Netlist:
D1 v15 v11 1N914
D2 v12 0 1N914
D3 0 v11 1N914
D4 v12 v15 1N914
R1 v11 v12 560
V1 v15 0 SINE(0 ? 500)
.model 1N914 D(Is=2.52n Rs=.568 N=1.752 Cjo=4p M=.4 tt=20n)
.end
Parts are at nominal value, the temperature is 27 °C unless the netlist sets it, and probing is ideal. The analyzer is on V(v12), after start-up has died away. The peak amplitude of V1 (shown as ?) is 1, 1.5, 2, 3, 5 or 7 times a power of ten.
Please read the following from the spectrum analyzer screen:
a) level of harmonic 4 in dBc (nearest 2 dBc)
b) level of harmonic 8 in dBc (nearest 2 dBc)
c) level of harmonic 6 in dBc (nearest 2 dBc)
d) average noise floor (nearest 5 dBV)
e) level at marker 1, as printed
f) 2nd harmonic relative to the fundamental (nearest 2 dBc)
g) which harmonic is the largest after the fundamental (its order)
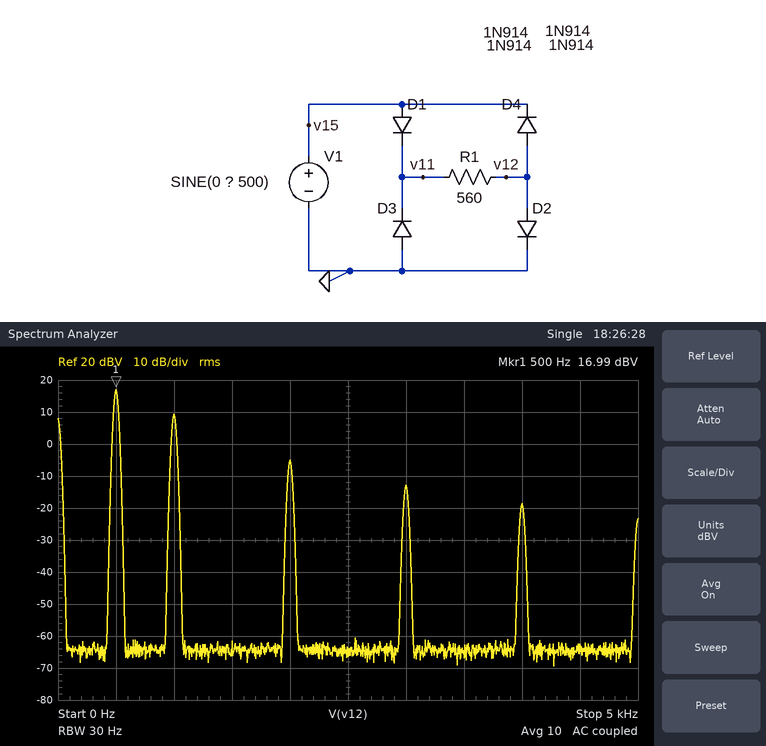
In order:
-22 dBc
-36 dBc
-30 dBc
-65 dBV
16.99 dBV
-8 dBc
2
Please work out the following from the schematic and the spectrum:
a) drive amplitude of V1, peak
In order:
20 V
